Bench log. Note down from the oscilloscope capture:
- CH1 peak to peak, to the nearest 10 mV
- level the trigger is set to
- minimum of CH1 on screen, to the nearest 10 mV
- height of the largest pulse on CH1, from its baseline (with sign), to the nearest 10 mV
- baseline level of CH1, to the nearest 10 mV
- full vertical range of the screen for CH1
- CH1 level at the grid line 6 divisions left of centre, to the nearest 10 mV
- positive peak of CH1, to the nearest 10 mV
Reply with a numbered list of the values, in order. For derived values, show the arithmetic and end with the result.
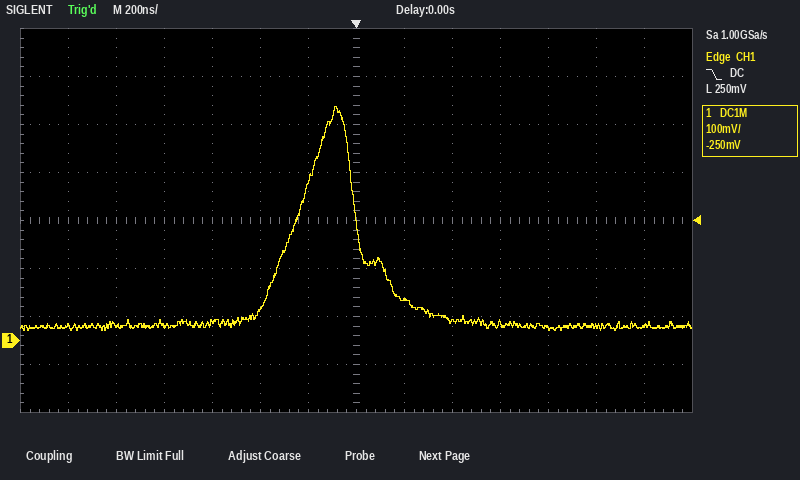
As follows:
1. 490 mV − (20 mV) = 470 mV
2. 250 mV
3. 20 mV
4. 490 mV − (30 mV) = +460 mV
5. 30 mV
6. 800 mV
7. 30 mV
8. 490 mV
